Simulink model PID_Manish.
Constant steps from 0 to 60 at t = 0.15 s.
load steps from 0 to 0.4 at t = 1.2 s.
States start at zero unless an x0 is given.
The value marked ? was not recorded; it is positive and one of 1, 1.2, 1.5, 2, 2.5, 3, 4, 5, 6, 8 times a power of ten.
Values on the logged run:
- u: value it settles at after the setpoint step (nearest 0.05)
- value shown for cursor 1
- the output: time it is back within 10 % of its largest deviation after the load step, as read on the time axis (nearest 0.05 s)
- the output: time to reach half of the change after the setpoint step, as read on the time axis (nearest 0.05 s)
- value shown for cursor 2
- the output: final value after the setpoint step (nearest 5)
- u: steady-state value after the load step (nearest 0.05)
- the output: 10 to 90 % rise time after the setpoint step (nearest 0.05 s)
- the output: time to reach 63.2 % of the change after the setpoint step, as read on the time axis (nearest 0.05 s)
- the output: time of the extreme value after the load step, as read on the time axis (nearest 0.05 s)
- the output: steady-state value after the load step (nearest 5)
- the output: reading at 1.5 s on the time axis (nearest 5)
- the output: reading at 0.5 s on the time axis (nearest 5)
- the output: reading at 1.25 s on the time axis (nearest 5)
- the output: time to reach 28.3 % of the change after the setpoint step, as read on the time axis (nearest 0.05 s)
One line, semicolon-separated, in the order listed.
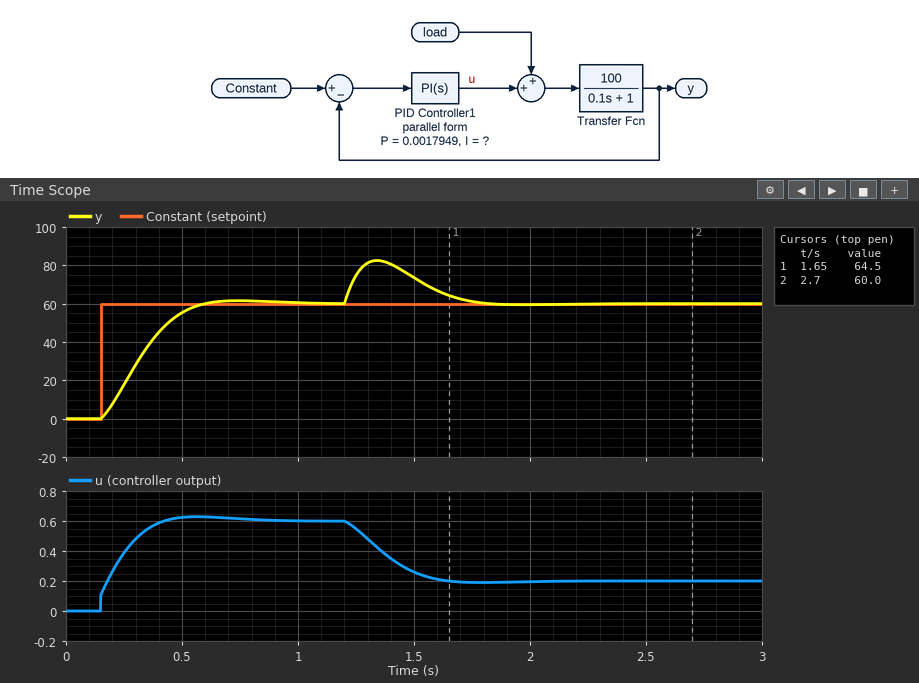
0.60; 64.5; 1.70 s; 0.30 s; 60.0; 60; 0.20; 0.30 s; 0.35 s; 1.35 s; 60; 75; 55; 75; 0.25 s
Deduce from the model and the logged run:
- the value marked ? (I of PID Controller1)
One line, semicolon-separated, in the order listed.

0.06
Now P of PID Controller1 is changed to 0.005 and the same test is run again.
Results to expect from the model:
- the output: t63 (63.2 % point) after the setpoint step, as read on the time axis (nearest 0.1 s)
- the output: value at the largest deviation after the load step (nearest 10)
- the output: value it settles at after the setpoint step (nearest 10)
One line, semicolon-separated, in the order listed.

0.3 s; 80; 60
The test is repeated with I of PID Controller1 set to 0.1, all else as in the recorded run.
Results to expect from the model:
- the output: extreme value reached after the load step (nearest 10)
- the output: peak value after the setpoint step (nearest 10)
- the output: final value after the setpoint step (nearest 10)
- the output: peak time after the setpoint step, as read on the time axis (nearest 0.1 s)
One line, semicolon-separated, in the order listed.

80; 70; 60; 0.5 s
